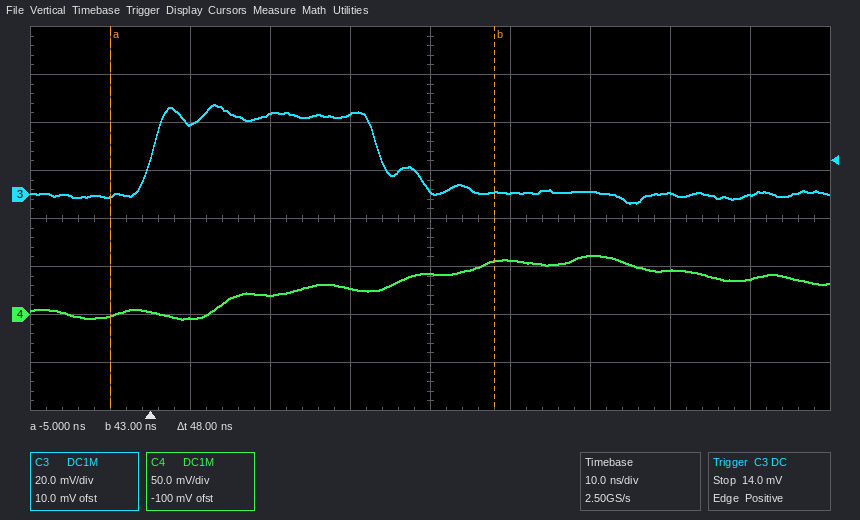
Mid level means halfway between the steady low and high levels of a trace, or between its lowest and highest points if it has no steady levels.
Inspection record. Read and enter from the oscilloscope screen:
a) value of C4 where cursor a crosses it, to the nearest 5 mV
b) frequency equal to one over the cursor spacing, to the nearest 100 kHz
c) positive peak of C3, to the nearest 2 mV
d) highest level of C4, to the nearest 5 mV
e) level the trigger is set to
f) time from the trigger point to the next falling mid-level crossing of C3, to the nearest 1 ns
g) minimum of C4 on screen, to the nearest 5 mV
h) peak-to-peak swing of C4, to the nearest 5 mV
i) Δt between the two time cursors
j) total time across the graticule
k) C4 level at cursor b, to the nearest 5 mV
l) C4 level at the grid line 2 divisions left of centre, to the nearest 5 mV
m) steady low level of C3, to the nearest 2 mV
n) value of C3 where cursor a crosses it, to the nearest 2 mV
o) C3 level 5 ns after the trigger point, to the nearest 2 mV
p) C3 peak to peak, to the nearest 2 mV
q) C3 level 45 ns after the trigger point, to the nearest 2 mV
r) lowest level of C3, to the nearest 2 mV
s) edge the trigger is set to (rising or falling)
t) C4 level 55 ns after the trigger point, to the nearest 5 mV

0 mV
20.8 MHz
38 mV
60 mV
14.0 mV
29 ns
-5 mV
65 mV
48 ns
100 ns
55 mV
20 mV
0 mV
0 mV
30 mV
42 mV
0 mV
-4 mV
rising
60 mV
